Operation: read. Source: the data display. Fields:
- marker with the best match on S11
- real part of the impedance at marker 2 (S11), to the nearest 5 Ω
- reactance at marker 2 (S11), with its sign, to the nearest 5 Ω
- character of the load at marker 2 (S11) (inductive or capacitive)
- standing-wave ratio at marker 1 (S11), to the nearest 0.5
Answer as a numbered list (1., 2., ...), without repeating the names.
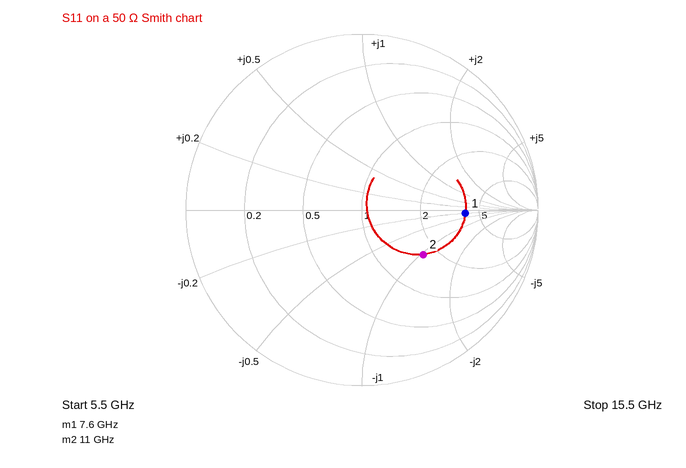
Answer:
1. marker 2
2. 85 Ω
3. -50 Ω
4. capacitive
5. 4.0
